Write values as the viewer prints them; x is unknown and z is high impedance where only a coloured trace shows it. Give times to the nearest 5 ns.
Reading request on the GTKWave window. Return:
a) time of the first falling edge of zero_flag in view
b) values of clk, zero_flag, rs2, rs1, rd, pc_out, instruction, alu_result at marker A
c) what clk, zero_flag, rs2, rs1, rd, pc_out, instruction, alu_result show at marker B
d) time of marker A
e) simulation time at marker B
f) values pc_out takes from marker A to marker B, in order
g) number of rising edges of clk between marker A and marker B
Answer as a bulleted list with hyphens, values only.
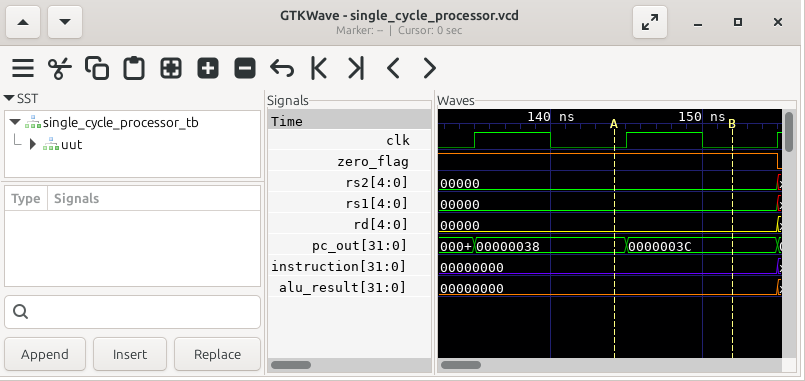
- 155 ns
- clk=0, zero_flag=1, rs2=00000, rs1=00000, rd=00000, pc_out=00000038, instruction=00000000, alu_result=00000000
- clk=0, zero_flag=1, rs2=00000, rs1=00000, rd=00000, pc_out=0000003C, instruction=00000000, alu_result=00000000
- 145 ns
- 150 ns
- 00000038, 0000003C
- 1
